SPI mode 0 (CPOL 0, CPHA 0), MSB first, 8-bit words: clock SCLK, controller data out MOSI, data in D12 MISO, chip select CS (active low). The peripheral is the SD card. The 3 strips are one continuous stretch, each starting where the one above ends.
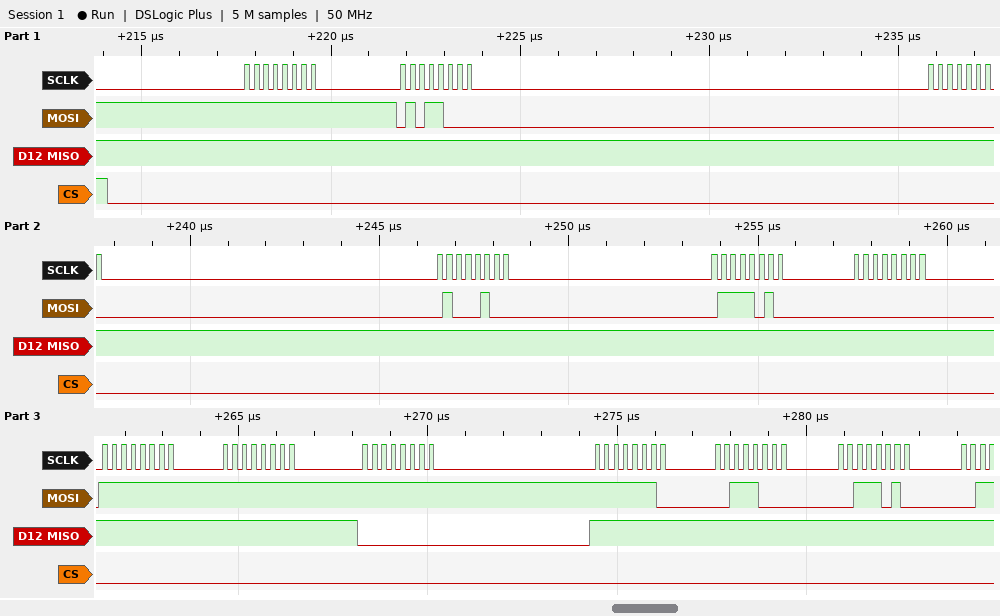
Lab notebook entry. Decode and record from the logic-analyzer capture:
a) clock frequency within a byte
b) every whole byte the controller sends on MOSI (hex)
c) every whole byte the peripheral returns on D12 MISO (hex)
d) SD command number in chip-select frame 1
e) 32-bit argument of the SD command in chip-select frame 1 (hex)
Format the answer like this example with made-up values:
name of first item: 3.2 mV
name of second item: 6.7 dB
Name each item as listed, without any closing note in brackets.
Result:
clock frequency within a byte: 4 MHz
every whole byte the controller sends on MOSI: FF 58 00 44 7A 00 FF FF FF FE 38 3A
every whole byte the peripheral returns on D12 MISO: FF FF FF FF FF FF FF FF 00 FF FF FF
SD command number in chip-select frame 1: CMD24
32-bit argument of the SD command in chip-select frame 1: 0x00447A00
